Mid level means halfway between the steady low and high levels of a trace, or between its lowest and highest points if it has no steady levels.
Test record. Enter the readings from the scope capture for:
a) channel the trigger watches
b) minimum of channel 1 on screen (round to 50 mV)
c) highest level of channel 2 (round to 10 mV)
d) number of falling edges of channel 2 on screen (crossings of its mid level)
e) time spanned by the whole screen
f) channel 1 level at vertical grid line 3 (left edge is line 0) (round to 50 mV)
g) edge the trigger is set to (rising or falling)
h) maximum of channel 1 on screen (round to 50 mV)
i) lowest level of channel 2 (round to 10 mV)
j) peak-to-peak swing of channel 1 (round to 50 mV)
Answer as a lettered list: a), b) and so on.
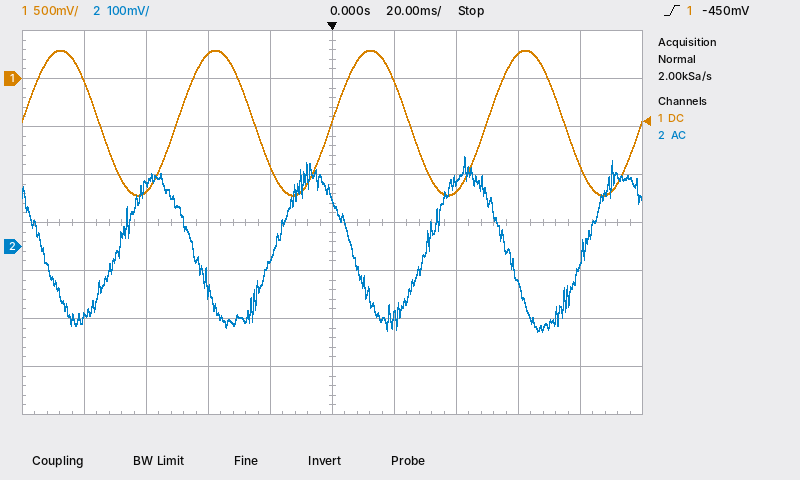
a) channel 1
b) -1.20 V
c) 190 mV
d) 4
e) 200 ms
f) 250 mV
g) rising
h) 300 mV
i) -180 mV
j) 1.50 V
